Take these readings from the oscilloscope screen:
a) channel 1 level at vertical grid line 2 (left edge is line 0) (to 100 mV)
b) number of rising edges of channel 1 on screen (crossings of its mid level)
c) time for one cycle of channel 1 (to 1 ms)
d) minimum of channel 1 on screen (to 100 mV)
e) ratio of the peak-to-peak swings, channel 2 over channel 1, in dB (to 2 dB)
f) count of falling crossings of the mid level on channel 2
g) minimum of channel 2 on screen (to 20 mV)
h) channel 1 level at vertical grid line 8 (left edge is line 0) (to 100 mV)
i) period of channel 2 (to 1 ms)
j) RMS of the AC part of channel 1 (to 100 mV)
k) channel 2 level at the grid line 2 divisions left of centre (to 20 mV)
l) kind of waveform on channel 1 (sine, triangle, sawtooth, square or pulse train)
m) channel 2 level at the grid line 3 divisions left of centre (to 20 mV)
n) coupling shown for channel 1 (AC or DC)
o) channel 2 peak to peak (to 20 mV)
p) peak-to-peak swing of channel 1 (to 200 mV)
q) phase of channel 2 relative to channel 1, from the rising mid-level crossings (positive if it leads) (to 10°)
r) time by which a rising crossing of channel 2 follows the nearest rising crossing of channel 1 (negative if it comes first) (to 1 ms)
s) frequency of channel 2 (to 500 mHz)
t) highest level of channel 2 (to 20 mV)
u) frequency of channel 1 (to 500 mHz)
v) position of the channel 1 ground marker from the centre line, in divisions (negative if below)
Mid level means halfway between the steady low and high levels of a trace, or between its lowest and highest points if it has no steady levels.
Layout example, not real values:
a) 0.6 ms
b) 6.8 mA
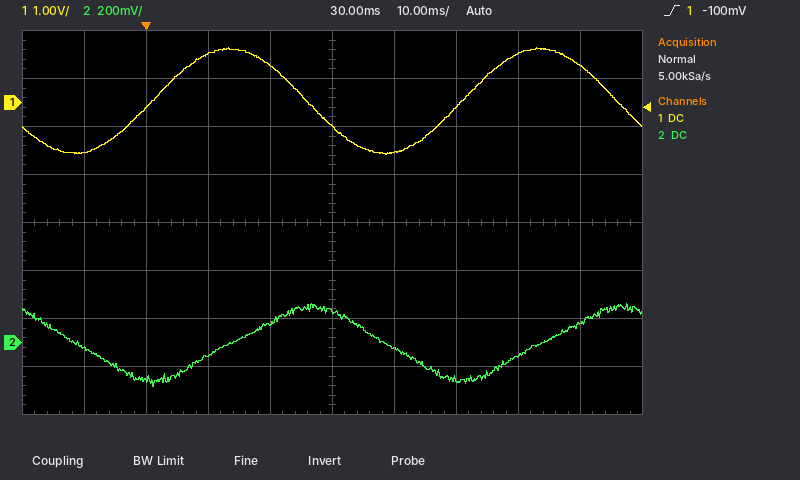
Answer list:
a) -100 mV
b) 2
c) 50 ms
d) -1.1 V
e) -16 dB
f) 2
g) -180 mV
h) 1.0 V
i) 50 ms
j) 800 mV
k) -60 mV
l) sine
m) -160 mV
n) DC
o) 340 mV
p) 2.2 V
q) -90°
r) +12 ms
s) 20.0 Hz
t) 160 mV
u) 20.0 Hz
v) +2.5 div
